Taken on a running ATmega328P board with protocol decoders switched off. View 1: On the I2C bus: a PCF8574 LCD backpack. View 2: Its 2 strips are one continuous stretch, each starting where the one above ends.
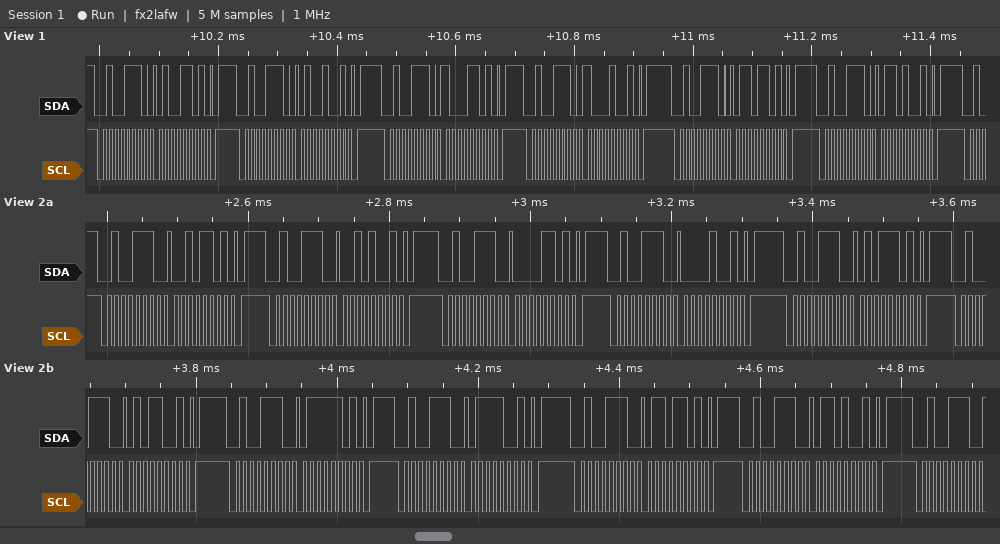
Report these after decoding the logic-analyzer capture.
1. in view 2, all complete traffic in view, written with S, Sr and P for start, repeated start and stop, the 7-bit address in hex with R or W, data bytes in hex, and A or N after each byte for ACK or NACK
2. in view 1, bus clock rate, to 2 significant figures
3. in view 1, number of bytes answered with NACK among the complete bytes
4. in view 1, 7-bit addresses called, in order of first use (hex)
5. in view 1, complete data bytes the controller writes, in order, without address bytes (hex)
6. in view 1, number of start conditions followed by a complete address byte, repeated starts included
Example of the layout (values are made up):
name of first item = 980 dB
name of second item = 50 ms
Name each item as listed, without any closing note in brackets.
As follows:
in view 2, all complete traffic in view, written with S, Sr and P for start, repeated start and stop, the 7-bit address in hex with R or W, data bytes in hex, and A or N after each byte for ACK or NACK = S 27W A 2D A P S 27W A 29 A P S 27W A 0D A P S 27W A 09 A P S 27W A 5D A P S 27W A 59 A P S 27W A 7D A P S 27W A 79 A P S 27W A 6D A P S 27W A 69 A P S 27W A
in view 1, bus clock rate, to 2 significant figures = 100 kHz
in view 1, number of bytes answered with NACK among the complete bytes = 0
in view 1, 7-bit addresses called, in order of first use = 0x27
in view 1, complete data bytes the controller writes, in order, without address bytes = 4D 49 8D 89 6D 69
in view 1, number of start conditions followed by a complete address byte, repeated starts included = 6
